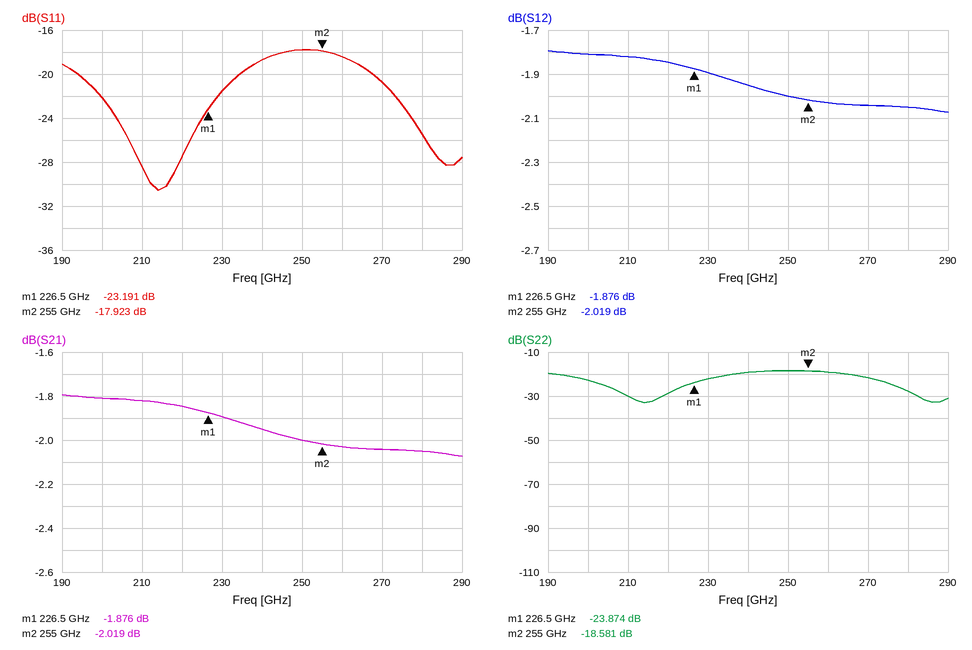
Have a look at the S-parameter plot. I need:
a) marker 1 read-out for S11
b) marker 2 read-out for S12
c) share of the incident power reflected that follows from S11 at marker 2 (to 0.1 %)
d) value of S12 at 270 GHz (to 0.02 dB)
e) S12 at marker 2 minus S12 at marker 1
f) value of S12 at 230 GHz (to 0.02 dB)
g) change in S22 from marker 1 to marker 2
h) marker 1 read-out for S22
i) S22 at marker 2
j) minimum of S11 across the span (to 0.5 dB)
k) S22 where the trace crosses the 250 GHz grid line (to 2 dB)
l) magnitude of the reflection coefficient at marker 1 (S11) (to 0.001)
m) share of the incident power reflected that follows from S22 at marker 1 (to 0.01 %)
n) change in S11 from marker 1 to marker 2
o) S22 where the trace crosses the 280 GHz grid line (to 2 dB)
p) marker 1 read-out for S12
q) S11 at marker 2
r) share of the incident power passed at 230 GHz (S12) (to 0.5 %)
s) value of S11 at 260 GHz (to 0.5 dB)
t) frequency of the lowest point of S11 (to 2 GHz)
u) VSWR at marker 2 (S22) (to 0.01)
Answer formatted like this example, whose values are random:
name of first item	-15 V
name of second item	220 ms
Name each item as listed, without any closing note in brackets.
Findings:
marker 1 read-out for S11	-23.191 dB
marker 2 read-out for S12	-2.019 dB
share of the incident power reflected that follows from S11 at marker 2	1.6 %
value of S12 at 270 GHz	-2.04 dB
S12 at marker 2 minus S12 at marker 1	-0.143 dB
value of S12 at 230 GHz	-1.90 dB
change in S22 from marker 1 to marker 2	5.293 dB
marker 1 read-out for S22	-23.874 dB
S22 at marker 2	-18.581 dB
minimum of S11 across the span	-30.5 dB
S22 where the trace crosses the 250 GHz grid line	-18 dB
magnitude of the reflection coefficient at marker 1 (S11)	0.069
share of the incident power reflected that follows from S22 at marker 1	0.41 %
change in S11 from marker 1 to marker 2	5.268 dB
S22 where the trace crosses the 280 GHz grid line	-28 dB
marker 1 read-out for S12	-1.876 dB
S11 at marker 2	-17.923 dB
share of the incident power passed at 230 GHz (S12)	64.5 %
value of S11 at 260 GHz	-18.5 dB
frequency of the lowest point of S11	214 GHz
VSWR at marker 2 (S22)	1.27
